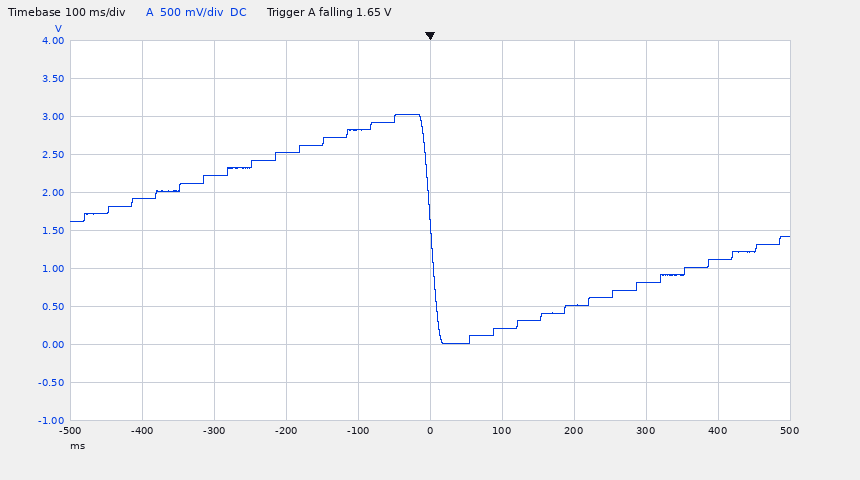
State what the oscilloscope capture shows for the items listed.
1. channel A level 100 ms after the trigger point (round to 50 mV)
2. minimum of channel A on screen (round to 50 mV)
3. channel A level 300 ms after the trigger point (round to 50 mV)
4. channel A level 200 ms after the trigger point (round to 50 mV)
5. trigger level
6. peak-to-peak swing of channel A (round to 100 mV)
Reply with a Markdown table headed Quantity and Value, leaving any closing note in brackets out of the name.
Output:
| Quantity | Value |
|---|---|
| channel A level 100 ms after the trigger point | 200 mV |
| minimum of channel A on screen | 0 mV |
| channel A level 300 ms after the trigger point | 800 mV |
| channel A level 200 ms after the trigger point | 500 mV |
| trigger level | 1.65 V |
| peak-to-peak swing of channel A | 3.00 V |
